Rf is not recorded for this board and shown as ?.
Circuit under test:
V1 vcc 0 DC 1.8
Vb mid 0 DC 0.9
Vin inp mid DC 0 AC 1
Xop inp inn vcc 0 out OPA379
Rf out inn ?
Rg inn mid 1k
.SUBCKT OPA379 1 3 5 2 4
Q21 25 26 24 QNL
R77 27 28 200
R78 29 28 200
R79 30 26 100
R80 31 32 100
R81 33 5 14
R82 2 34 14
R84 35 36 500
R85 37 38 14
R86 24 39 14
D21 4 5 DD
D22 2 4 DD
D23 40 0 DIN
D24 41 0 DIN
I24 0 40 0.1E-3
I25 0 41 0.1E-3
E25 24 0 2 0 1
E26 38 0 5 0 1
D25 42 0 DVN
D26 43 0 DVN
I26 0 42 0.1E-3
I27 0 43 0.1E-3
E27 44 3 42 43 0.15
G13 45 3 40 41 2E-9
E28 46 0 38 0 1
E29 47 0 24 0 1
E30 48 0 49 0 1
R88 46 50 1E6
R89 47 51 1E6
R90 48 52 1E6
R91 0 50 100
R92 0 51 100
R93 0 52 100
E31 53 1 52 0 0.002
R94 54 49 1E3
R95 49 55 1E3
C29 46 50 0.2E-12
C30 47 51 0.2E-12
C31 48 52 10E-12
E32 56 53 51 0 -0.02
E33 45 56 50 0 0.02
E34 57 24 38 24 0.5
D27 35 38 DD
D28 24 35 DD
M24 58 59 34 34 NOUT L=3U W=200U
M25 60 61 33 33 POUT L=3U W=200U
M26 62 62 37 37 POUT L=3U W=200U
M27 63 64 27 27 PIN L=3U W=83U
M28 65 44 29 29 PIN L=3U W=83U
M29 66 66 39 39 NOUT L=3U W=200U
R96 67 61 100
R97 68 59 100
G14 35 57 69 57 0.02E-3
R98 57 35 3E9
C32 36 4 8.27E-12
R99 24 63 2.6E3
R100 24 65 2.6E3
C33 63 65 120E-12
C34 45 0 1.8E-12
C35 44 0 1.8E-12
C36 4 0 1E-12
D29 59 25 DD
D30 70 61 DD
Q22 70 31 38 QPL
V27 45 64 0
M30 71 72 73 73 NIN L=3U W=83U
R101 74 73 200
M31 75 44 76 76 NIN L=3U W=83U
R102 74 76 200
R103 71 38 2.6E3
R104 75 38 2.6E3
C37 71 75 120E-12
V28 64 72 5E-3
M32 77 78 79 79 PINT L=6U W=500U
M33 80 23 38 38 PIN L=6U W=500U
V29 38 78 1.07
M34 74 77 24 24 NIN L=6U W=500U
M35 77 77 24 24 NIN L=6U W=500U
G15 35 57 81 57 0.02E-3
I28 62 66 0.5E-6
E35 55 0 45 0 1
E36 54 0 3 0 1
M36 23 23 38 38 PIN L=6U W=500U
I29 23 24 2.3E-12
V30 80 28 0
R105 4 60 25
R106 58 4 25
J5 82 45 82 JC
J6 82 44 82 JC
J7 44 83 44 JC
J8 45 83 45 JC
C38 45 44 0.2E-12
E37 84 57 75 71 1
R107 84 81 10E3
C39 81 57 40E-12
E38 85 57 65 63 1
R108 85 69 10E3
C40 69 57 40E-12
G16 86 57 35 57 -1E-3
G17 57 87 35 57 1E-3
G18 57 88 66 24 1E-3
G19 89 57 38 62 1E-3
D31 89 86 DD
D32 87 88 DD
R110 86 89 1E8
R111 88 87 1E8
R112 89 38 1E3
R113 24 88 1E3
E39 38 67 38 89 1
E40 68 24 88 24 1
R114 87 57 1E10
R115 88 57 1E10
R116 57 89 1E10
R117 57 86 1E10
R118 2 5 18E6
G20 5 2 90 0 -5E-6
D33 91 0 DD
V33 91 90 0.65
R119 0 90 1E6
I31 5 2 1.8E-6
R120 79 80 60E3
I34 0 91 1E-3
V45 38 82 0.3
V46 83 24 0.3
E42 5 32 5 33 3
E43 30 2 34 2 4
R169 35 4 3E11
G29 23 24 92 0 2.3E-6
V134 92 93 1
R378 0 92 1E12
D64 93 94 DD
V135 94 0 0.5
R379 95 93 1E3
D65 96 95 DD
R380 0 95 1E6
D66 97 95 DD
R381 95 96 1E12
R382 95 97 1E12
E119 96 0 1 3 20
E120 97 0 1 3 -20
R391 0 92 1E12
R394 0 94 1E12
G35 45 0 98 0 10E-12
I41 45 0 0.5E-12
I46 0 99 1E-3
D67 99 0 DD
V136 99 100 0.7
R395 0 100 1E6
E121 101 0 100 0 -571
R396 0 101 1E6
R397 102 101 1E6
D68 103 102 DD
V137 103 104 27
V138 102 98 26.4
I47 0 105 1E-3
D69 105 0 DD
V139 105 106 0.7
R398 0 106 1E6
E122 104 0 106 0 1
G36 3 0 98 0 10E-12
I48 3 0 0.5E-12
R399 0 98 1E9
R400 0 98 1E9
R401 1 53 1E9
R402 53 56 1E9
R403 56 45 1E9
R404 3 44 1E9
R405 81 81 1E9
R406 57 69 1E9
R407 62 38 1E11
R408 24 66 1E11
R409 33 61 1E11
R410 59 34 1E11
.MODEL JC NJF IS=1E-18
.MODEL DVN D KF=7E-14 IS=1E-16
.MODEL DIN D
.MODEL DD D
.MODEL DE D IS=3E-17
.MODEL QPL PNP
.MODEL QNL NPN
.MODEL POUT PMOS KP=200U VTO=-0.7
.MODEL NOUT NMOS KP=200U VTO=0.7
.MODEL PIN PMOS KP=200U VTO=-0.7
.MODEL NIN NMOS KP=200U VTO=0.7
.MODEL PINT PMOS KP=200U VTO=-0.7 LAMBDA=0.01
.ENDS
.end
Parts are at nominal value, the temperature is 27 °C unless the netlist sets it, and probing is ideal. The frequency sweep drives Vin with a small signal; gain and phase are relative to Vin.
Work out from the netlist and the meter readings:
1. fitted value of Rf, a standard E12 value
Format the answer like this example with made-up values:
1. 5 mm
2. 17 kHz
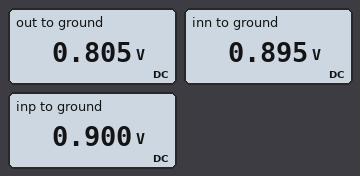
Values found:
1. 18 kΩ
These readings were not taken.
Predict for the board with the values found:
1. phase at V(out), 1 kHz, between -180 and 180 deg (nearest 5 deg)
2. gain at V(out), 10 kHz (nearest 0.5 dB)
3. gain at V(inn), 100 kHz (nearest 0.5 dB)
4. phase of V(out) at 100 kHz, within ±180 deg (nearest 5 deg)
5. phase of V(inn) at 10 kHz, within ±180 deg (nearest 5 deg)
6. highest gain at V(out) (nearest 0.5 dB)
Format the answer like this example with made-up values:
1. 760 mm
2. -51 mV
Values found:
1. -10 deg
2. 19.0 dB
3. -26.5 dB
4. -125 deg
5. -65 deg
6. 25.5 dB
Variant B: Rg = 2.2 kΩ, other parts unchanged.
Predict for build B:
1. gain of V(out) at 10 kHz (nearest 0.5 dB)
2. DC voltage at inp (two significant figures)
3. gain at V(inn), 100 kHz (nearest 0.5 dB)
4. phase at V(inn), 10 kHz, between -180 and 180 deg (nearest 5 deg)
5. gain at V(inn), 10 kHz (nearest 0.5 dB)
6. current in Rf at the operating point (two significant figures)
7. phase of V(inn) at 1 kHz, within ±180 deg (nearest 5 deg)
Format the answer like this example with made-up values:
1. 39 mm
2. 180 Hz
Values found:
1. 16.5 dB
2. 900 mV
3. -20.5 dB
4. -45 deg
5. -2.5 dB
6. 2.3 µA
7. -5 deg
